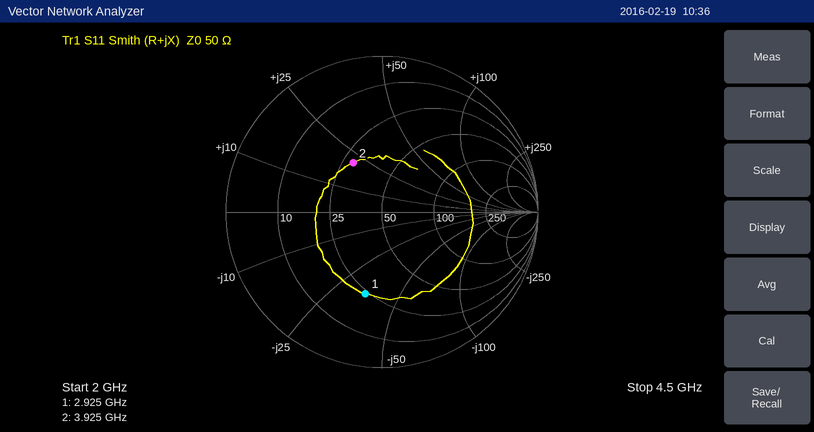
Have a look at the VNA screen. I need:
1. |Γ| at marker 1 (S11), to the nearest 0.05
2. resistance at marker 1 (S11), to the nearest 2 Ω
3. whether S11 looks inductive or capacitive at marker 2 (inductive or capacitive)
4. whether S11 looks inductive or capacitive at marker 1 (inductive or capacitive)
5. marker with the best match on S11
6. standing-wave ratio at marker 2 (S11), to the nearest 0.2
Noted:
0.55
24 Ω
inductive
capacitive
marker 2
2.2
